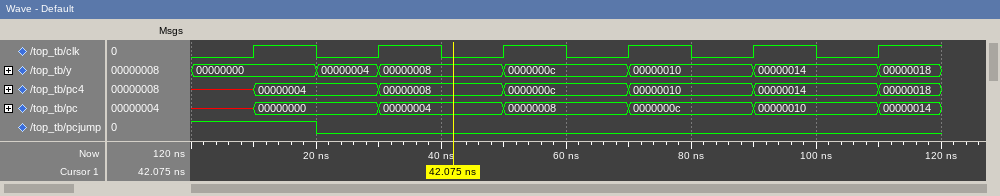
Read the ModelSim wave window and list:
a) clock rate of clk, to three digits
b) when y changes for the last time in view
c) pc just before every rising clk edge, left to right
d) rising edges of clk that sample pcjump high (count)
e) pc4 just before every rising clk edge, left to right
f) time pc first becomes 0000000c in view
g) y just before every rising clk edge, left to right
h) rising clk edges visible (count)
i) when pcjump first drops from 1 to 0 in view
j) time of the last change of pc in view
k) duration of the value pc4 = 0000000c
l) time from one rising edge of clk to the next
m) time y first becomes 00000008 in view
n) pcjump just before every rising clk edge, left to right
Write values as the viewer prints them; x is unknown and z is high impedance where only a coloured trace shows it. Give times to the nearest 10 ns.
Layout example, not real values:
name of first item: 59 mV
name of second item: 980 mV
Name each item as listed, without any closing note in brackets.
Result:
clock rate of clk, to three digits: 50.0 MHz
when y changes for the last time in view: 110 ns
pc just before every rising clk edge, left to right: x, 00000000, 00000004, 00000008, 0000000c, 00000010
rising edges of clk that sample pcjump high: 1
pc4 just before every rising clk edge, left to right: x, 00000004, 00000008, 0000000c, 00000010, 00000014
time pc first becomes 0000000c in view: 70 ns
y just before every rising clk edge, left to right: 00000000, 00000004, 00000008, 0000000c, 00000010, 00000014
rising clk edges visible: 6
when pcjump first drops from 1 to 0 in view: 20 ns
time of the last change of pc in view: 110 ns
duration of the value pc4 = 0000000c: 20 ns
time from one rising edge of clk to the next: 20 ns
time y first becomes 00000008 in view: 30 ns
pcjump just before every rising clk edge, left to right: 1 0 0 0 0 0
